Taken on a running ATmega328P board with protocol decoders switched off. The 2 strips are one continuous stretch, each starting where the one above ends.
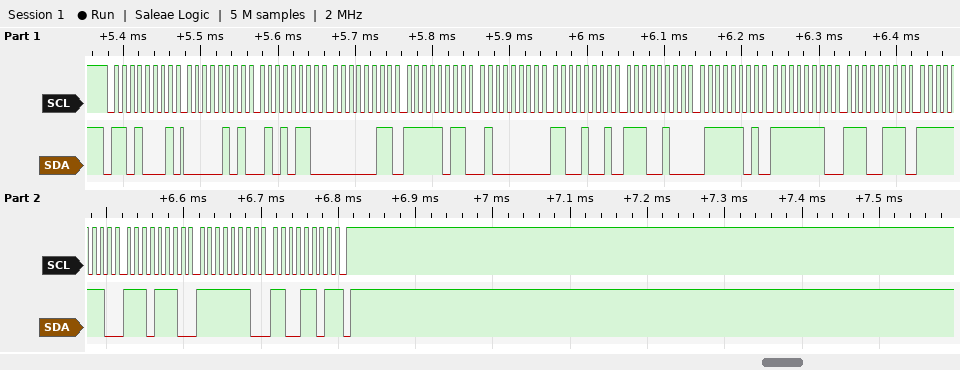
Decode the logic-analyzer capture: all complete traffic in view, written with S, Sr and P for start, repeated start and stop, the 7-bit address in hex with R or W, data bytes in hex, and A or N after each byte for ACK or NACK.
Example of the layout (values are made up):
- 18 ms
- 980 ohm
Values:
- S 68R A 05 A 56 A 03 A FB A 40 A C9 A E4 A 7D A FE A E7 A FE A EE A FE A CD N P
